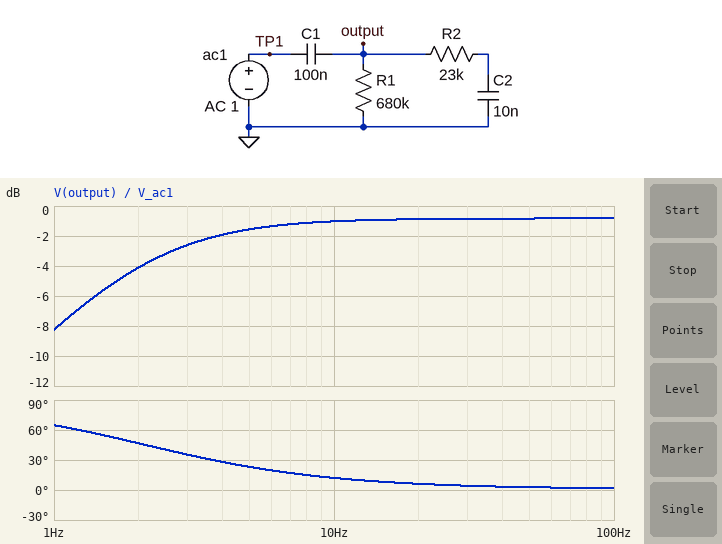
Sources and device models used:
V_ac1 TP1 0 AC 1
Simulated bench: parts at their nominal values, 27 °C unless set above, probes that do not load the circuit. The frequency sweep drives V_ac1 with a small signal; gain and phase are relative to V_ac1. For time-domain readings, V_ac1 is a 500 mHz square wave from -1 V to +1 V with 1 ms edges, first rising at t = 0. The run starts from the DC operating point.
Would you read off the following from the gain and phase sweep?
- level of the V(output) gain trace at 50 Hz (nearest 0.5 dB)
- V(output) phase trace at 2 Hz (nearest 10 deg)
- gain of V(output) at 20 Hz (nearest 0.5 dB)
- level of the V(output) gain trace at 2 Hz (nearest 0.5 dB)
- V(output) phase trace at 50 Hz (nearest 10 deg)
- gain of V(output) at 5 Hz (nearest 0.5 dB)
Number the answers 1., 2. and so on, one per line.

1. -1.0 dB
2. 50 deg
3. -1.0 dB
4. -4.0 dB
5. 0 deg
6. -1.5 dB
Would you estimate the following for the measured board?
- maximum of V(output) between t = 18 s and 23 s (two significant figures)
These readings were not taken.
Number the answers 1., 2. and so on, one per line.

1. 1.8 V
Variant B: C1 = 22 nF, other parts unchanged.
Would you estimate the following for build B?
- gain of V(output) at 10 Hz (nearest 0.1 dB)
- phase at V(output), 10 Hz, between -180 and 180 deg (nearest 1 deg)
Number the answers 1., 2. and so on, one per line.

1. -5.1 dB
2. 36 deg
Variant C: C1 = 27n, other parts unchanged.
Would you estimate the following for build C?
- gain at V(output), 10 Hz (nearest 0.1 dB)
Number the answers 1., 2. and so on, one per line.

1. -4.2 dB
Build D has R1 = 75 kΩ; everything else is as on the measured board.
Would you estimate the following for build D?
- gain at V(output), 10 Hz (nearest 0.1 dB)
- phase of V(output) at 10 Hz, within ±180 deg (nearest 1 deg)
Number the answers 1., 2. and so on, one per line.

1. -7.6 dB
2. 63 deg
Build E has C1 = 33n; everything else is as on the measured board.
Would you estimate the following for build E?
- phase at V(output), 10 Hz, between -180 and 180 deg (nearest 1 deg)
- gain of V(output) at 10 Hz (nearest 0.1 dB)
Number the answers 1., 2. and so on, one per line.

1. 29 deg
2. -3.4 dB
